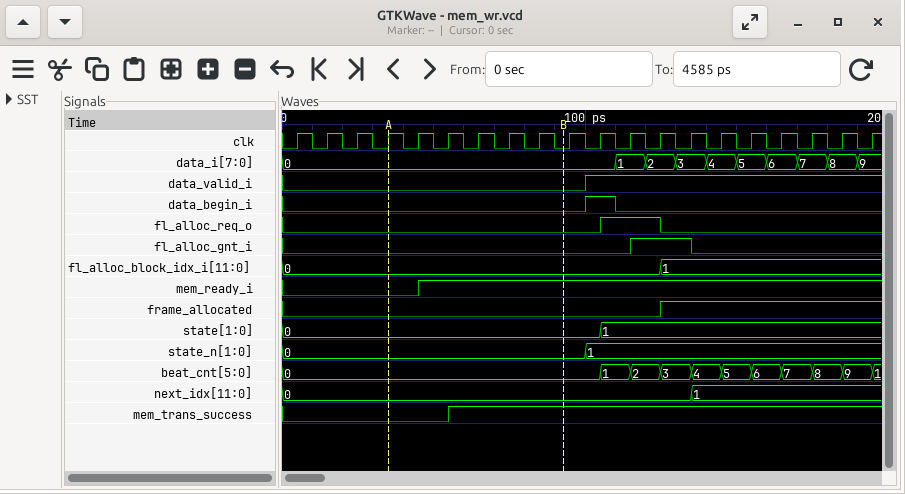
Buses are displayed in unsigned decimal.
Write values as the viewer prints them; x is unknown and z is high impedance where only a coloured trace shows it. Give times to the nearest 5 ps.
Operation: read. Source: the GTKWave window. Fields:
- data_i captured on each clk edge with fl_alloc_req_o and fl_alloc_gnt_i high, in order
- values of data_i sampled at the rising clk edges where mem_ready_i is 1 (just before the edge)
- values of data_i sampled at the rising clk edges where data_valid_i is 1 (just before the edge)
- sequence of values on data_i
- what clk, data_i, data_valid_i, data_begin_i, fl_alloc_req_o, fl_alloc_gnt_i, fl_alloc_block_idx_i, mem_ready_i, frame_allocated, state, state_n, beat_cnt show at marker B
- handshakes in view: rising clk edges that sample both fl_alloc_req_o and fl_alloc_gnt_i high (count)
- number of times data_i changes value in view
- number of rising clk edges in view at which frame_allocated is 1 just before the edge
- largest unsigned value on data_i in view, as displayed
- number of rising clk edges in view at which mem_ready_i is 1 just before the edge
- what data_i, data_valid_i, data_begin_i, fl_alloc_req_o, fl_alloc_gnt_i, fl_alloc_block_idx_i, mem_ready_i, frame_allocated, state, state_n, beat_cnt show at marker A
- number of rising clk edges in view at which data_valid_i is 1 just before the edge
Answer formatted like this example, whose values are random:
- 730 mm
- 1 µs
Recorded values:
- 2
- 0, 0, 0, 0, 0, 0, 1, 2, 3, 4, 5, 6, 7, 8, 9
- 0, 1, 2, 3, 4, 5, 6, 7, 8, 9
- 0, 1, 2, 3, 4, 5, 6, 7, 8, 9
- clk=0, data_i=0, data_valid_i=0, data_begin_i=0, fl_alloc_req_o=0, fl_alloc_gnt_i=0, fl_alloc_block_idx_i=0, mem_ready_i=1, frame_allocated=0, state=0, state_n=0, beat_cnt=0
- 1
- 9
- 7
- 9
- 15
- data_i=0, data_valid_i=0, data_begin_i=0, fl_alloc_req_o=0, fl_alloc_gnt_i=0, fl_alloc_block_idx_i=0, mem_ready_i=0, frame_allocated=0, state=0, state_n=0, beat_cnt=0
- 10
